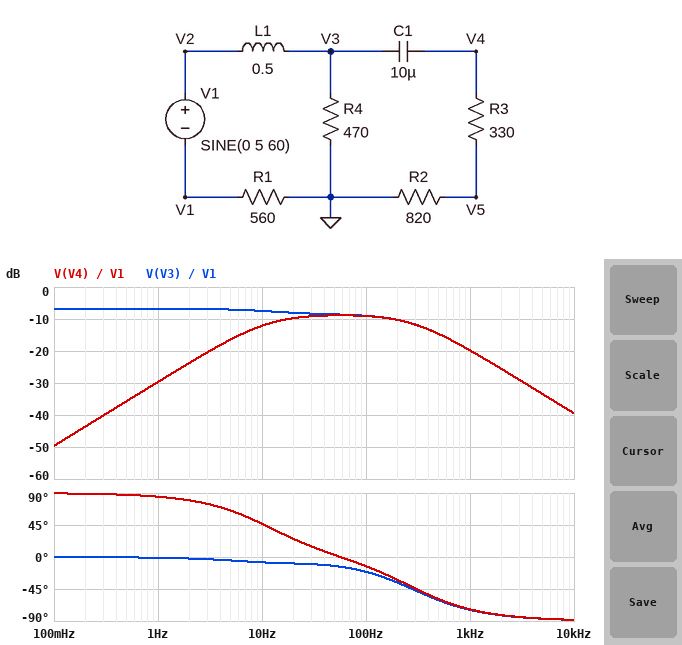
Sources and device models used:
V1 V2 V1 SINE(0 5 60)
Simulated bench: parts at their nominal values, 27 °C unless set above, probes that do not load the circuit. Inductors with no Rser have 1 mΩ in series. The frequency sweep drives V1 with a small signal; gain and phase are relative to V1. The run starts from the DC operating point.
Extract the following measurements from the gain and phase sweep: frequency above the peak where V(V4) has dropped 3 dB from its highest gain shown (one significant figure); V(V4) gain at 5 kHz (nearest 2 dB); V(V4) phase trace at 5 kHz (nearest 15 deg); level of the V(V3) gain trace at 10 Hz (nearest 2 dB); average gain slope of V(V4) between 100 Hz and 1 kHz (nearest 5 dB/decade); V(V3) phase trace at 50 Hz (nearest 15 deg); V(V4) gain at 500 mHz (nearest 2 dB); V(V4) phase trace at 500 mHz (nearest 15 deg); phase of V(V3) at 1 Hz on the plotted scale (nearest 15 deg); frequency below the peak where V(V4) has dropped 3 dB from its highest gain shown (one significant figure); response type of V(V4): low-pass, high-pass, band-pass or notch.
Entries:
300 Hz
-34 dB
-90 deg
-8 dB
-10 dB/decade
-15 deg
-36 dB
90 deg
0 deg
10 Hz
band-pass
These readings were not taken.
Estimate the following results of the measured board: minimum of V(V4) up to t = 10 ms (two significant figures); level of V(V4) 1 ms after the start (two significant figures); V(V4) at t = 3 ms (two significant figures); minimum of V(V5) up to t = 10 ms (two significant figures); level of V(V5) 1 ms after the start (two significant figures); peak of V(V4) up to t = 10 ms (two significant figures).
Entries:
-1.2 V
360 mV
1.3 V
-860 mV
260 mV
1.5 V
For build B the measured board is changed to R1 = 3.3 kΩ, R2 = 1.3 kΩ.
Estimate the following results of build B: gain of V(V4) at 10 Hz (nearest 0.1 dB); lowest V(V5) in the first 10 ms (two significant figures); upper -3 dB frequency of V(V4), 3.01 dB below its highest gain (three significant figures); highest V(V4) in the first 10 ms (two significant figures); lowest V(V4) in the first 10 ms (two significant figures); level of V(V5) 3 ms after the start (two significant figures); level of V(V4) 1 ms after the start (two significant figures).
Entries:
-22.1 dB
-290 mV
1.18 kHz
440 mV
-360 mV
320 mV
160 mV
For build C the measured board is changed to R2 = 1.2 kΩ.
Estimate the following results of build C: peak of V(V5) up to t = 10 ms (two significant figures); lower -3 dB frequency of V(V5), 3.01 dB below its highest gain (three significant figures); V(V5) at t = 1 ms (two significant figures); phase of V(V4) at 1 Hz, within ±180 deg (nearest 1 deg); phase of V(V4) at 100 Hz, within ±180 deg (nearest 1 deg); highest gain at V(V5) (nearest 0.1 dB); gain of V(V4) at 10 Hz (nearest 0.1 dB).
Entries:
1.3 V
8.44 Hz
300 mV
83 deg
-14 deg
-10.5 dB
-10.7 dB
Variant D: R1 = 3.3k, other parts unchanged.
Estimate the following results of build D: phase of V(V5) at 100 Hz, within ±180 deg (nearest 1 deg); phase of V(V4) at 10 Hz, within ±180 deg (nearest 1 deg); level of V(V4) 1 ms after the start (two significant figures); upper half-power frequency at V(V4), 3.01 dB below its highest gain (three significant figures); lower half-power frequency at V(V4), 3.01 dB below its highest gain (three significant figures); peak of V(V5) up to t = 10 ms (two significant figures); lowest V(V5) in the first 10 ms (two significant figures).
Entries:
1 deg
45 deg
140 mV
1.18 kHz
10.0 Hz
280 mV
-250 mV
